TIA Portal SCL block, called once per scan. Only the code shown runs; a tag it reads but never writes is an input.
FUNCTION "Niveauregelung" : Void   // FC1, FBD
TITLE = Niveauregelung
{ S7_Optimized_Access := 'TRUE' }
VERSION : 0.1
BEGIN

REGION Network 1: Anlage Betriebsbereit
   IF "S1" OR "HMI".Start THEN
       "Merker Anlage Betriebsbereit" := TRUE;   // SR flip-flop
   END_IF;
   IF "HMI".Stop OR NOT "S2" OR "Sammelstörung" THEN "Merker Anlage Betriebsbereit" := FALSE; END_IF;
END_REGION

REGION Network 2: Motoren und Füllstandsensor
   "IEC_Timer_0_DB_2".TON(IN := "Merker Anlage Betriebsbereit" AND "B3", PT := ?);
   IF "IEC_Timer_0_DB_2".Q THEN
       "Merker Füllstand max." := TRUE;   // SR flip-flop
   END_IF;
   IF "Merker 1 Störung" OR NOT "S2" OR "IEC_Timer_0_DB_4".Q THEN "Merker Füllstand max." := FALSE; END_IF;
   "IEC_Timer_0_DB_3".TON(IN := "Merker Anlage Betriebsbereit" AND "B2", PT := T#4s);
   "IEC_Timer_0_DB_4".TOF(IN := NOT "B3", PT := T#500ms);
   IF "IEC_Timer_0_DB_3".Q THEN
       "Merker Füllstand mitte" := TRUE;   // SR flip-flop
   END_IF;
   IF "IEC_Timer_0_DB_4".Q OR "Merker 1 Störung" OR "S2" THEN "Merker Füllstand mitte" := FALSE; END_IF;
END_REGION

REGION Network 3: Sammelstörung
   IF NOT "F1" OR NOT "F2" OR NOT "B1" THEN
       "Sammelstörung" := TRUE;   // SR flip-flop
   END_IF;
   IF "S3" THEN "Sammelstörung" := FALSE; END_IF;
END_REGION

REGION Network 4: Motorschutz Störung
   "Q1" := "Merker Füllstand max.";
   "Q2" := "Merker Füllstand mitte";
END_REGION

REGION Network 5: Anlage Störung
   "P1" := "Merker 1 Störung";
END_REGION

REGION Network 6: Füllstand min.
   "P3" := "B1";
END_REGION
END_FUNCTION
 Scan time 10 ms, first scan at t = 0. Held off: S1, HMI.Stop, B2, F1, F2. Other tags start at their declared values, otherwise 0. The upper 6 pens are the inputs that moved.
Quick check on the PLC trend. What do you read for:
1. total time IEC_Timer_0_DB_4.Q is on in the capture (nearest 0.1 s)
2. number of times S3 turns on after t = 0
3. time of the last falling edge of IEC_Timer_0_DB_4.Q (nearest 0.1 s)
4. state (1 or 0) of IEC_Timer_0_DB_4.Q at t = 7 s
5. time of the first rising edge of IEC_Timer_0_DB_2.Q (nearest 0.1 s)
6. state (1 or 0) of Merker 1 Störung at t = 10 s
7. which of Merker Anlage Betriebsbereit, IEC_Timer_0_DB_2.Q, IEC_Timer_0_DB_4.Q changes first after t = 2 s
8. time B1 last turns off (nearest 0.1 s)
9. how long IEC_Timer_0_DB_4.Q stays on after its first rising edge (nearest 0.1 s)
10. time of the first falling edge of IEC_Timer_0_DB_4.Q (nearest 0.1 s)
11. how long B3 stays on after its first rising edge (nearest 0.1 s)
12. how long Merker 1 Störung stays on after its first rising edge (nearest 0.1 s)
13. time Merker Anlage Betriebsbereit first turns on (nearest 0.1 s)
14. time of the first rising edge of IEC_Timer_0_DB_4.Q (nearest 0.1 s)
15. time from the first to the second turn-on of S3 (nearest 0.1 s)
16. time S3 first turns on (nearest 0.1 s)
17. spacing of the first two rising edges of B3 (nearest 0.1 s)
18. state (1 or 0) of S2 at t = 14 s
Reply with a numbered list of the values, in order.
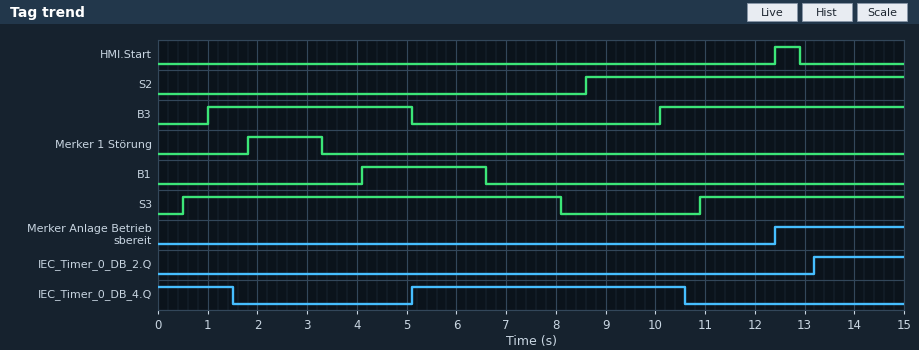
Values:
1. 7.0 s
2. 2
3. 10.6 s
4. 1
5. 13.2 s
6. 0
7. IEC_Timer_0_DB_4.Q
8. 6.6 s
9. 5.5 s
10. 1.5 s
11. 4.1 s
12. 1.5 s
13. 12.4 s
14. 5.1 s
15. 10.4 s
16. 0.5 s
17. 9.1 s
18. 1
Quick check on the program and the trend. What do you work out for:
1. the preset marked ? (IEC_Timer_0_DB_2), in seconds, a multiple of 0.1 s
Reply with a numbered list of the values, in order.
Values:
1. 0.8 s
